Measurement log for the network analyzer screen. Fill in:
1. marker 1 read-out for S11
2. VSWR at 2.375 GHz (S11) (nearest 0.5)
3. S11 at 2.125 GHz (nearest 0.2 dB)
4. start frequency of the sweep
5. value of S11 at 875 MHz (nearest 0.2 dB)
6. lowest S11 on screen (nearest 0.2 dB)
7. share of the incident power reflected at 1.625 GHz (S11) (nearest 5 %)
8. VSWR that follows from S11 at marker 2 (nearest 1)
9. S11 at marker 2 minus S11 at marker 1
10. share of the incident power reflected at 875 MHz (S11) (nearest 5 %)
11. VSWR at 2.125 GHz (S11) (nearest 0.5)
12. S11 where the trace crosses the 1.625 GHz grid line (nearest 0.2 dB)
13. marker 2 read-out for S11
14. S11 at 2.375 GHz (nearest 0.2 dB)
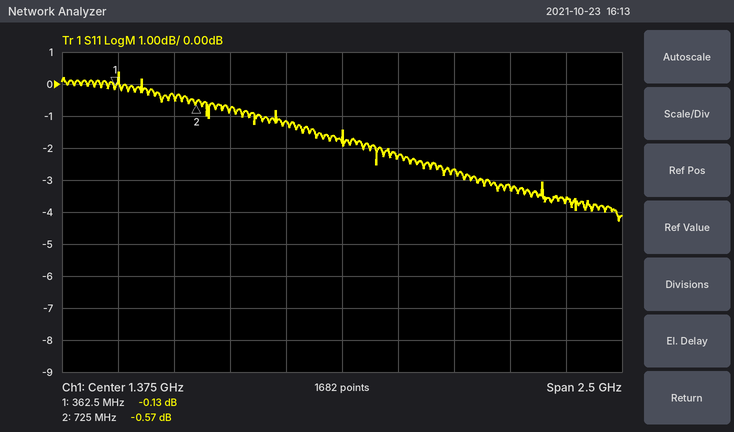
-0.13 dB
5.0
-3.2 dB
125 MHz
-0.8 dB
-4.2 dB
60 %
30
-0.44 dB
85 %
5.5
-2.2 dB
-0.57 dB
-3.6 dB
